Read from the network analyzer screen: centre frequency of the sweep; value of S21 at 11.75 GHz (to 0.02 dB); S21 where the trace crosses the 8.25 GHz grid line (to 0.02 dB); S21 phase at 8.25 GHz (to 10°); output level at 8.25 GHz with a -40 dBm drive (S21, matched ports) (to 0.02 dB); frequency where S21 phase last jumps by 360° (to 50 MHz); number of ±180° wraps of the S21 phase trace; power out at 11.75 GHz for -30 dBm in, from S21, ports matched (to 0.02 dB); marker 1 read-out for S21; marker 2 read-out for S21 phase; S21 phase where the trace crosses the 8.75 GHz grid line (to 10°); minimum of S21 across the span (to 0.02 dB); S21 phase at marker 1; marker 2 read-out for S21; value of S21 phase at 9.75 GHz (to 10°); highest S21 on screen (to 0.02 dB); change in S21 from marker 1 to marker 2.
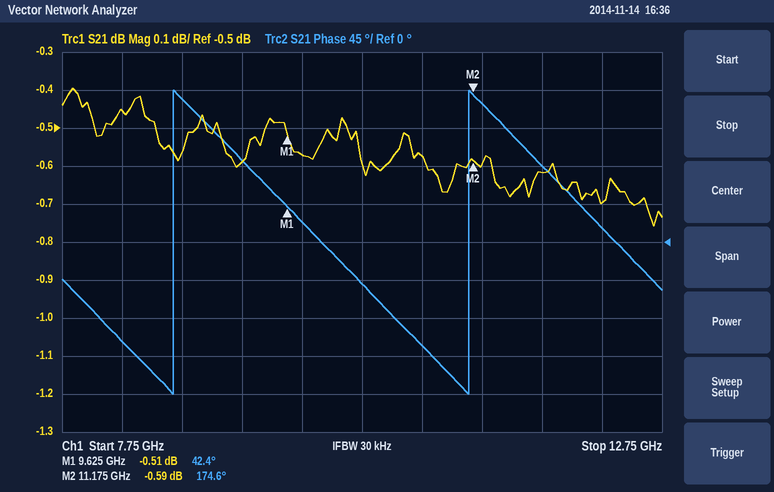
10.25 GHz
-0.62 dB
-0.46 dB
-120°
-40.46 dBm
11.15 GHz
2
-30.62 dBm
-0.51 dB
174.6°
170°
-0.76 dB
42.4°
-0.59 dB
20°
-0.40 dB
-0.08 dB
